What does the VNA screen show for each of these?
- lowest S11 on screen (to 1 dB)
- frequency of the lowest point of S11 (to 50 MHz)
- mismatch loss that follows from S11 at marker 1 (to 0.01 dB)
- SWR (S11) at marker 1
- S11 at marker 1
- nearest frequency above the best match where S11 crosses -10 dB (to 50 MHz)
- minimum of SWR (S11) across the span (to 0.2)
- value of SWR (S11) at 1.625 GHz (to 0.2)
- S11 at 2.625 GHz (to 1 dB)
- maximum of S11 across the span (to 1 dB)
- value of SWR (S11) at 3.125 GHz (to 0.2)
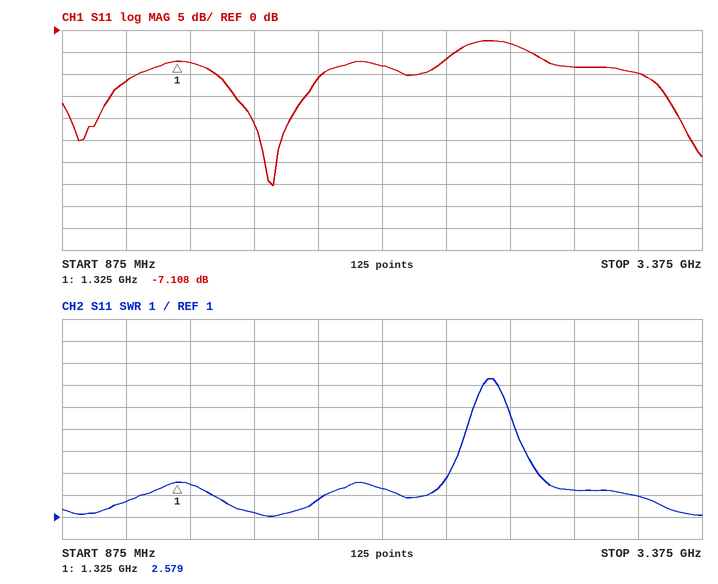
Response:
-35 dB
1.70 GHz
0.94 dB
2.579
-7.108 dB
1.90 GHz
1.0
1.2
-3 dB
-2 dB
2.0
